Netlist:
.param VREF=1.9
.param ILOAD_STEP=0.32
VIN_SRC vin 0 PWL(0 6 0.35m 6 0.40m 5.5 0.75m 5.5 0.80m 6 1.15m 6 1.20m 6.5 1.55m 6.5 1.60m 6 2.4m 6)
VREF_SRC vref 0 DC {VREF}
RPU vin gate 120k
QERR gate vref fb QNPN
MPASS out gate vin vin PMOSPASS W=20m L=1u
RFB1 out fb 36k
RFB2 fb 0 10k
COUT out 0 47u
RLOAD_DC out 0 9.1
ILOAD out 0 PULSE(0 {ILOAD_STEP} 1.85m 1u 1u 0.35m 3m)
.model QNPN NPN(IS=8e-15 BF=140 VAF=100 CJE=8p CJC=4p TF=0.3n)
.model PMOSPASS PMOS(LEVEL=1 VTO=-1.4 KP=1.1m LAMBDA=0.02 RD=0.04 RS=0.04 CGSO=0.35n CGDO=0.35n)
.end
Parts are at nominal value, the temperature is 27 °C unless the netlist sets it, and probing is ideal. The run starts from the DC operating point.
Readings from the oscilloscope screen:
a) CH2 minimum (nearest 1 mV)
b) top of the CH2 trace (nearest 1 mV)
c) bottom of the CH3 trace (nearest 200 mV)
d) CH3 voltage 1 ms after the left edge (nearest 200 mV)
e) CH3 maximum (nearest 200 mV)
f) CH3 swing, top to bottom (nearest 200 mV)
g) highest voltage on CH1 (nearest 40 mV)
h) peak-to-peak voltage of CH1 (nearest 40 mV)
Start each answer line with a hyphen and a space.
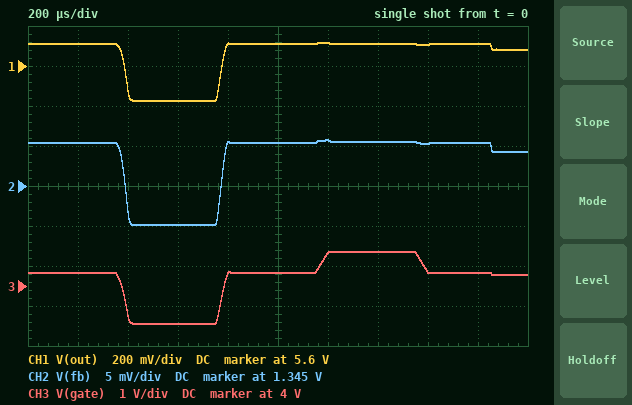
- 1.340 V
- 1.351 V
- 3.0 V
- 4.4 V
- 4.8 V
- 1.8 V
- 5.72 V
- 280 mV
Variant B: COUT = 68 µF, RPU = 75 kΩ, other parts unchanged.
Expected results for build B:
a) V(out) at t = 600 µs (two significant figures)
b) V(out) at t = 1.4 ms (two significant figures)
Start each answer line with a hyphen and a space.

- 5.3 V
- 5.4 V
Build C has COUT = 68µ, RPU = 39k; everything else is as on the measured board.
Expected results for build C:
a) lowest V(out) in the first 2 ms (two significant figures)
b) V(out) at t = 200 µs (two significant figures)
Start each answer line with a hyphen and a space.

- 4.5 V
- 4.6 V
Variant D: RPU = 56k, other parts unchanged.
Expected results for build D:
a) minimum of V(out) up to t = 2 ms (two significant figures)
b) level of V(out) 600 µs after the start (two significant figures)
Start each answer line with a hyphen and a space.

- 5.0 V
- 5.1 V
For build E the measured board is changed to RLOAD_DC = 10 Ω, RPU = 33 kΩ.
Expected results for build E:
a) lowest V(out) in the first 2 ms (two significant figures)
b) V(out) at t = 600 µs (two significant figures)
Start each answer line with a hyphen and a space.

- 4.2 V
- 4.3 V
